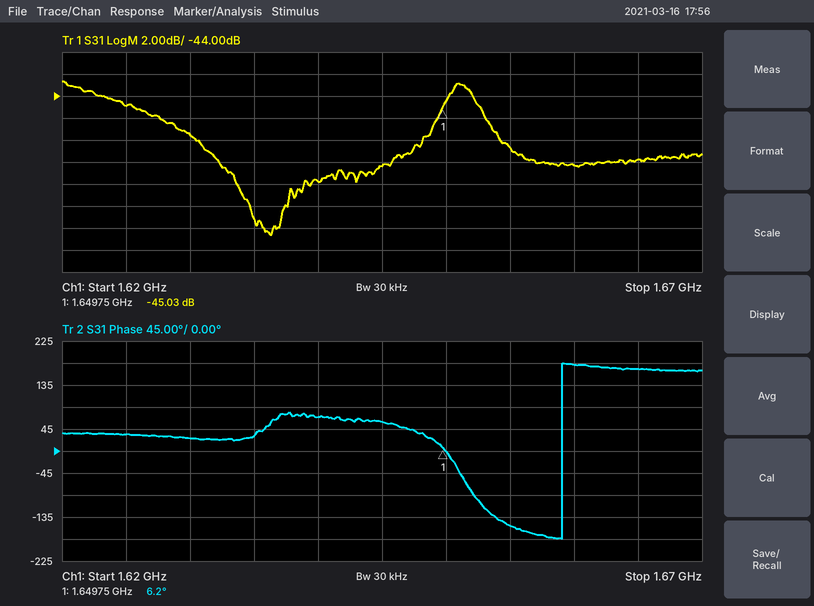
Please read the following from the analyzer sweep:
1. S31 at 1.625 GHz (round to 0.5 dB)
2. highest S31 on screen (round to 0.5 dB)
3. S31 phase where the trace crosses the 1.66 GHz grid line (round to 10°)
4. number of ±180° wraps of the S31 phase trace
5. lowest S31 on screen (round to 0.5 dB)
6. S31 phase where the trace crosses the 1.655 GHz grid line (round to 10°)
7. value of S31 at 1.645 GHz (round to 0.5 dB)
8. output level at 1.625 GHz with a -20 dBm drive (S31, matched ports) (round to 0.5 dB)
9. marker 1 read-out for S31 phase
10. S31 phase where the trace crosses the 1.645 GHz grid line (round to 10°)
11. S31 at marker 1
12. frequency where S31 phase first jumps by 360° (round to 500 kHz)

-45.0 dB
-42.5 dB
180°
1
-56.5 dB
-150°
-50.5 dB
-65.0 dBm
6.2°
60°
-45.03 dB
1.6590 GHz
